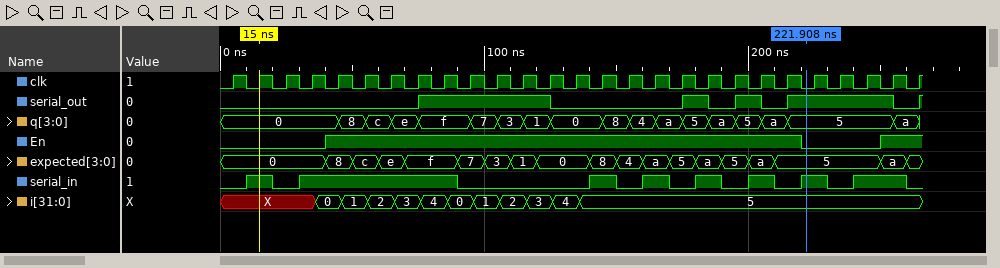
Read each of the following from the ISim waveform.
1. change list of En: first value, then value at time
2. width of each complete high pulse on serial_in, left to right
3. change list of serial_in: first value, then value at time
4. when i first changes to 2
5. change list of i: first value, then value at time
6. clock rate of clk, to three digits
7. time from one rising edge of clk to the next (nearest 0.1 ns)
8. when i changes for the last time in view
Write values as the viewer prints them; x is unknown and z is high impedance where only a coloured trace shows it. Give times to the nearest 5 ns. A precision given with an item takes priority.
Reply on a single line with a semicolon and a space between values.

0, 1 at 40 ns, 0 at 220 ns, 1 at 250 ns; 10 ns, 60 ns, 10 ns, 10 ns, 10 ns, 10 ns, 10 ns, 20 ns; 0, 1 at 10 ns, 0 at 20 ns, 1 at 30 ns, 0 at 90 ns, 1 at 140 ns, 0 at 150 ns, 1 at 160 ns, 0 at 170 ns, 1 at 180 ns, 0 at 190 ns, 1 at 200 ns, 0 at 210 ns, 1 at 220 ns, 0 at 230 ns, 1 at 240 ns, 0 at 260 ns; 55 ns; X, 0 at 35 ns, 1 at 45 ns, 2 at 55 ns, 3 at 65 ns, 4 at 75 ns, 0 at 85 ns, 1 at 95 ns, 2 at 105 ns, 3 at 115 ns, 4 at 125 ns, 5 at 135 ns; 100 MHz; 10 ns; 135 ns
